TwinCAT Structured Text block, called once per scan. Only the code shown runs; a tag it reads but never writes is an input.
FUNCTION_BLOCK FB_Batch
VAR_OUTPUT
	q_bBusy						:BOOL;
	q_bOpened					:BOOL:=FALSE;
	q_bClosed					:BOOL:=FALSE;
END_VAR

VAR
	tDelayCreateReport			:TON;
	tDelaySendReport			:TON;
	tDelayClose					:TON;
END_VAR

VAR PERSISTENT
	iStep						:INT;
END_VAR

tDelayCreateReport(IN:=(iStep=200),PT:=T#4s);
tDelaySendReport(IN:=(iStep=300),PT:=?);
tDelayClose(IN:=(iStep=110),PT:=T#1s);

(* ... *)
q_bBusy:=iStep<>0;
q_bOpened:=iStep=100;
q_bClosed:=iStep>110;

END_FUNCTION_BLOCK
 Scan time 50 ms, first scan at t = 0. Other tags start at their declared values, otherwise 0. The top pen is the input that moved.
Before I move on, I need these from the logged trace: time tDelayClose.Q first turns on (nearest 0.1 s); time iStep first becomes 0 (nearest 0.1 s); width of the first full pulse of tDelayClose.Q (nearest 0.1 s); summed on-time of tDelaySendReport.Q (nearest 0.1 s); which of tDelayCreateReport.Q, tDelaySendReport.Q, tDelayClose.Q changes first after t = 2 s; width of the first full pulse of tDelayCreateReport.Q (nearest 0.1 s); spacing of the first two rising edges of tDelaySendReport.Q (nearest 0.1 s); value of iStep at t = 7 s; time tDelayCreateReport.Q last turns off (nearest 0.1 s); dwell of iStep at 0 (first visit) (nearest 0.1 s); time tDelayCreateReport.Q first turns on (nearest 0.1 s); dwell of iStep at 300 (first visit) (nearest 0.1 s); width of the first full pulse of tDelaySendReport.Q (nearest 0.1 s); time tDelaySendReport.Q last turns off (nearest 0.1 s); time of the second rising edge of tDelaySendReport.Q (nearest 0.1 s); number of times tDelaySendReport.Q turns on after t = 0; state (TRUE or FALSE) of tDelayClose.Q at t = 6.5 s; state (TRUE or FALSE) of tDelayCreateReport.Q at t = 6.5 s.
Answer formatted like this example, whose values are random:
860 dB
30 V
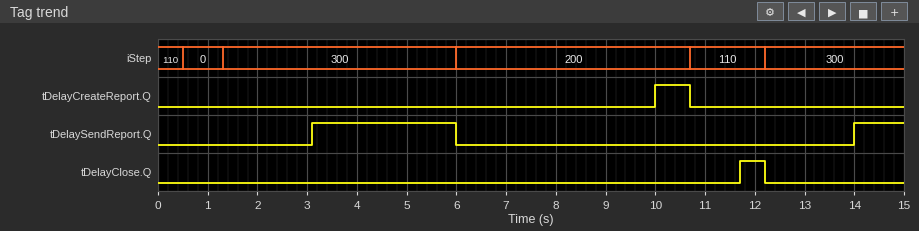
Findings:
11.7 s
0.5 s
0.5 s
3.9 s
tDelaySendReport.Q
0.7 s
10.9 s
200
10.7 s
0.8 s
10.0 s
4.7 s
2.9 s
6.0 s
14.0 s
2
FALSE
FALSE
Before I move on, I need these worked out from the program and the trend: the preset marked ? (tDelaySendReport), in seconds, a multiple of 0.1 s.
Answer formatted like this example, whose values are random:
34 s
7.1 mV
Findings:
1.8 s
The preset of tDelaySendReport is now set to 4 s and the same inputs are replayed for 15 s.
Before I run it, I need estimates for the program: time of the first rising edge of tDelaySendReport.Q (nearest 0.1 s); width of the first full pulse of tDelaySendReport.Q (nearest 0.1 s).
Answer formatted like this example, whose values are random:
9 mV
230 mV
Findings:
5.3 s
0.7 s
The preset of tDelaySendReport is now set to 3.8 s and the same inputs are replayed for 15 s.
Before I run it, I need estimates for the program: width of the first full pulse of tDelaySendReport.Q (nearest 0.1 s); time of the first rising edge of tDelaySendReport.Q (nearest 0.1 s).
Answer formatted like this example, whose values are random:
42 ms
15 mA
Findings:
0.9 s
5.1 s
